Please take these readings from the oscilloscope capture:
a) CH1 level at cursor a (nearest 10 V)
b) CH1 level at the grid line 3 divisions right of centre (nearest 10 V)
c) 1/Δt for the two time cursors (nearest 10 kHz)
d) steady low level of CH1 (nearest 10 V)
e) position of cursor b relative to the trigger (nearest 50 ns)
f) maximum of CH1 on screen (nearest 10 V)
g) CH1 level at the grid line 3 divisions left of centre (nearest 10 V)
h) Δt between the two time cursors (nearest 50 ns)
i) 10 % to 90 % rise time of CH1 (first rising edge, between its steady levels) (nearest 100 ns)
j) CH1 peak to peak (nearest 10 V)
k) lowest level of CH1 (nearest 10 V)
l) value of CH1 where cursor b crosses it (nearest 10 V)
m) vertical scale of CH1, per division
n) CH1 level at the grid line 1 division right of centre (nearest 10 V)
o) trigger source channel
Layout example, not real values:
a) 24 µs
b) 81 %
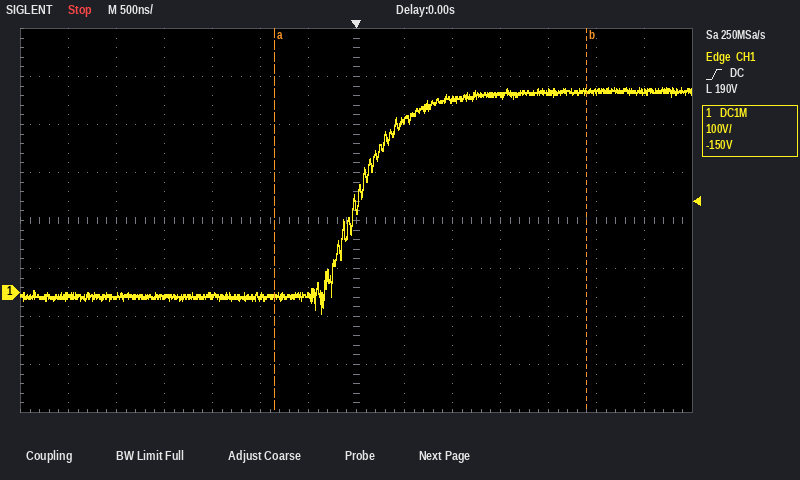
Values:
a) -10 V
b) 410 V
c) 310 kHz
d) -10 V
e) +2.40 µs
f) 430 V
g) -10 V
h) 3.25 µs
i) 900 ns
j) 470 V
k) -40 V
l) 420 V
m) 100 V
n) 360 V
o) CH1
